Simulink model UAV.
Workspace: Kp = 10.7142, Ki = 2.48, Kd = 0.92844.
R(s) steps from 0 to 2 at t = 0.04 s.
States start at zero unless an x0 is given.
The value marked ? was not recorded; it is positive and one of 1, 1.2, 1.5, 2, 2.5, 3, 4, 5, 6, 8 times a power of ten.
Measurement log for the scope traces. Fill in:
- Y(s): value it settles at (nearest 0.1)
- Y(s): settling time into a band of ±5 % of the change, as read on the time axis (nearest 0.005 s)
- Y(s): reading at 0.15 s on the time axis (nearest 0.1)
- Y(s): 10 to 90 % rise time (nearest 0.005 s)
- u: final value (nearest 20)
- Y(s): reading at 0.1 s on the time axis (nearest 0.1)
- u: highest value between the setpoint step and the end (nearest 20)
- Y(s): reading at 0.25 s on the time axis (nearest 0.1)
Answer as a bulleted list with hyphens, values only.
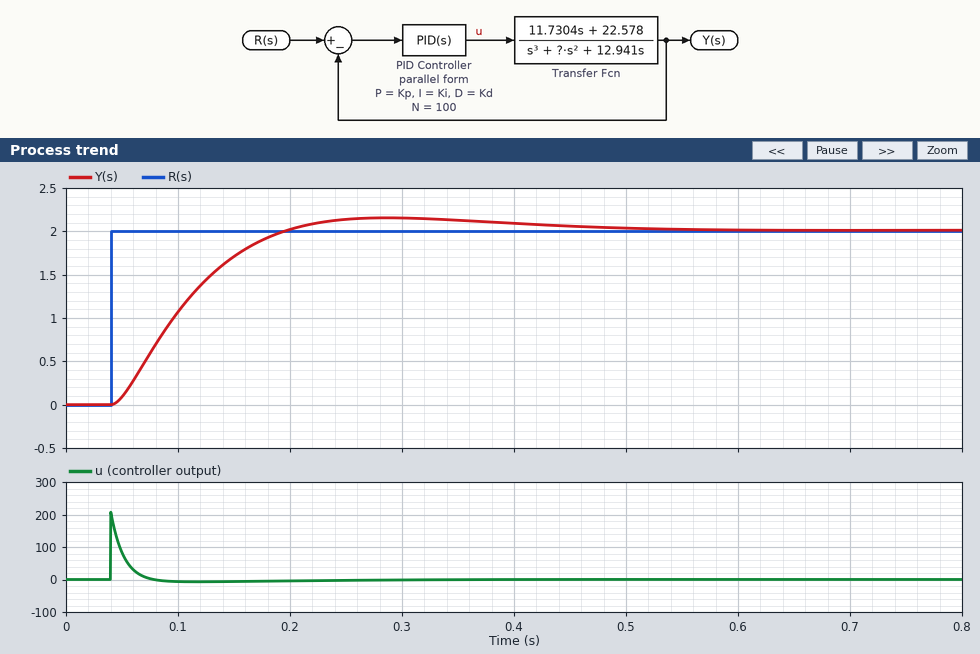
- 2.0
- 0.375 s
- 1.7
- 0.105 s
- 0
- 1.1
- 200
- 2.1
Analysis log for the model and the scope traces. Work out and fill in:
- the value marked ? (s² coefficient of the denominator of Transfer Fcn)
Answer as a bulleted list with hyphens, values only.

- 8
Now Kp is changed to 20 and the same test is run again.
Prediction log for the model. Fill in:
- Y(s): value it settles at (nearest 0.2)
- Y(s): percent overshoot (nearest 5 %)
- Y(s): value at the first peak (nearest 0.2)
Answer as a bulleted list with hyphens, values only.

- 2.0
- 20 %
- 2.4
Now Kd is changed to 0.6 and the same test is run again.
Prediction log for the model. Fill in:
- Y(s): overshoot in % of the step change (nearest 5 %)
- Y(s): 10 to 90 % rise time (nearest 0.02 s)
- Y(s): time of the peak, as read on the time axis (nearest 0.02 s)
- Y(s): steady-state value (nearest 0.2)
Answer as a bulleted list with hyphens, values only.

- 15 %
- 0.12 s
- 0.30 s
- 2.0
